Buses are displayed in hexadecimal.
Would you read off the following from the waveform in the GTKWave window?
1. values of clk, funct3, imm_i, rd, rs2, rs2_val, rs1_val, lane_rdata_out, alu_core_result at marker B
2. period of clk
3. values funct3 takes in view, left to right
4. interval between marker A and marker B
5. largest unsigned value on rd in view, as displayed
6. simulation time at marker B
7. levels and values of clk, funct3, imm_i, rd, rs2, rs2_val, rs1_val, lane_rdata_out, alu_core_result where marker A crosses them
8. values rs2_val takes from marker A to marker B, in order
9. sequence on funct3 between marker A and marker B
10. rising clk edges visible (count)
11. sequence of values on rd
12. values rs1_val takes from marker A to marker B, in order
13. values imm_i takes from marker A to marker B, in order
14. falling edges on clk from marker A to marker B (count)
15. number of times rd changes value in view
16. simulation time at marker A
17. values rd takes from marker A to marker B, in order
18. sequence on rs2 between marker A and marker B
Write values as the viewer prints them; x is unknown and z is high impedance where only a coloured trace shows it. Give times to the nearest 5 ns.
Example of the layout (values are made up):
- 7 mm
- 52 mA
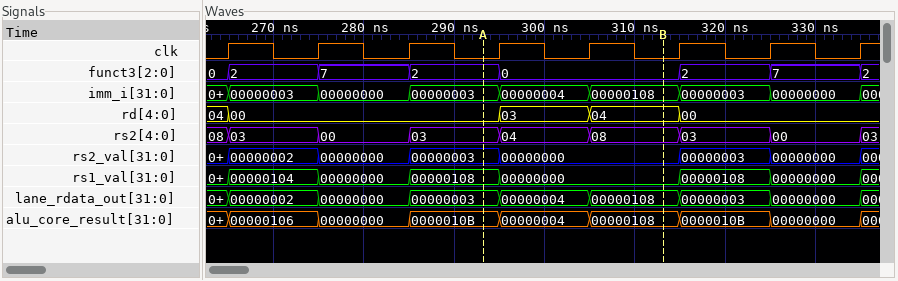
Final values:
- clk=0, funct3=0, imm_i=00000108, rd=04, rs2=08, rs2_val=00000000, rs1_val=00000000, lane_rdata_out=00000108, alu_core_result=00000108
- 10 ns
- 0, 2, 7, 2, 0, 2, 7, 2
- 20 ns
- 04
- 315 ns
- clk=0, funct3=2, imm_i=00000003, rd=00, rs2=03, rs2_val=00000003, rs1_val=00000108, lane_rdata_out=00000003, alu_core_result=0000010B
- 00000003, 00000000
- 2, 0
- 8
- 04, 00, 03, 04, 00
- 00000108, 00000000
- 00000003, 00000004, 00000108
- 2
- 4
- 295 ns
- 00, 03, 04
- 03, 04, 08
